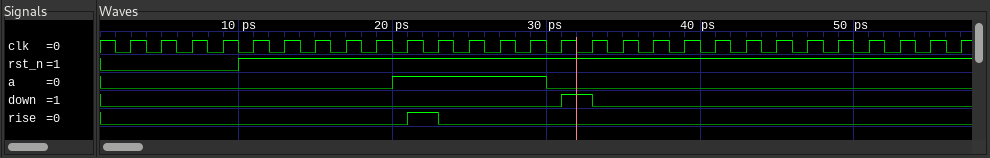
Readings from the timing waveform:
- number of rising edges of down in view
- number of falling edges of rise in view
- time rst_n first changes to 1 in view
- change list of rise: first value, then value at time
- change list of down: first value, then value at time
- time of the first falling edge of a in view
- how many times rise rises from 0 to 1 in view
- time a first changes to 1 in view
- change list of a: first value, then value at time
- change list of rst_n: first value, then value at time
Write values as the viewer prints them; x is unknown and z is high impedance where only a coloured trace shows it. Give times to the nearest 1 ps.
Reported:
1
1
10 ps
0, 1 at 21 ps, 0 at 23 ps
0, 1 at 31 ps, 0 at 33 ps
30 ps
1
20 ps
0, 1 at 20 ps, 0 at 30 ps
0, 1 at 10 ps
